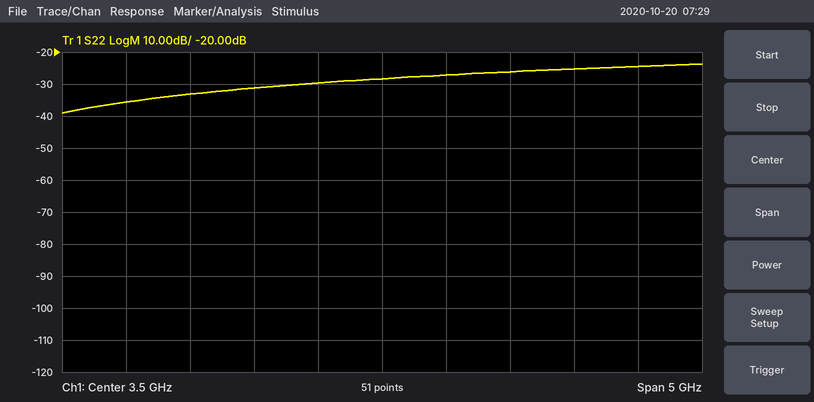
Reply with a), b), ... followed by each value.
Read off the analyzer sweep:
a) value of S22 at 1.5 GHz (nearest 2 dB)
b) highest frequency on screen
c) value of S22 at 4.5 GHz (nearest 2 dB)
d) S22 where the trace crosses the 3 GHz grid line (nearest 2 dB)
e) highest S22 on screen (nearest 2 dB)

a) -36 dB
b) 6 GHz
c) -26 dB
d) -30 dB
e) -24 dB
